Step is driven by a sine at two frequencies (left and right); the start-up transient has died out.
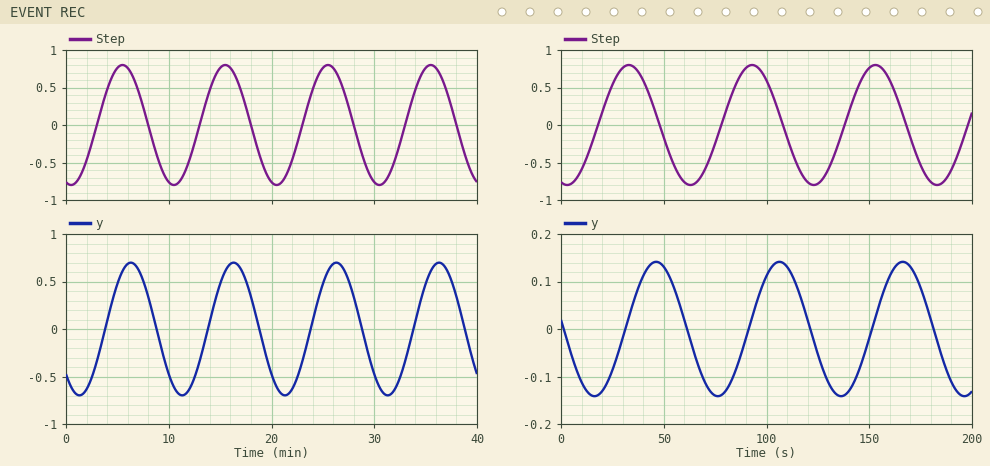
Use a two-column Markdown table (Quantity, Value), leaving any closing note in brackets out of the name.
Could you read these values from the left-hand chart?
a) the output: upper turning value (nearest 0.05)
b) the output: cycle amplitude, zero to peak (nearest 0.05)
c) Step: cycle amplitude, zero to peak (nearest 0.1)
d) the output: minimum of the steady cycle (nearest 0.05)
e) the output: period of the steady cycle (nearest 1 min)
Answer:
| Quantity | Value |
|---|---|
| the output: upper turning value | 0.70 |
| the output: cycle amplitude, zero to peak | 0.70 |
| Step: cycle amplitude, zero to peak | 0.8 |
| the output: minimum of the steady cycle | -0.70 |
| the output: period of the steady cycle | 10 min |
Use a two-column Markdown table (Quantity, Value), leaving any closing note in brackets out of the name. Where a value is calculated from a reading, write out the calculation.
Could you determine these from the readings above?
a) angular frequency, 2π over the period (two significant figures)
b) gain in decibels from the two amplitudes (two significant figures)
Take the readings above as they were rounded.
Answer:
| Quantity | Value |
|---|---|
| angular frequency, 2π over the period | 2π / 10 = 0.63 rad/min |
| gain in decibels from the two amplitudes | 20 log10(0.7 / 0.8) = -1.2 dB |
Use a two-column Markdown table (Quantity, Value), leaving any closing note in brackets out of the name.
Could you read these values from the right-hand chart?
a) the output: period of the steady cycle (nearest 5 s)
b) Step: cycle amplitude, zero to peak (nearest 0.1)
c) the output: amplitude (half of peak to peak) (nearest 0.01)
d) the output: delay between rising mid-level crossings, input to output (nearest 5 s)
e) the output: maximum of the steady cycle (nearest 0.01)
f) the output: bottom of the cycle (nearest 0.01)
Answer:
| Quantity | Value |
|---|---|
| the output: period of the steady cycle | 60 s |
| Step: cycle amplitude, zero to peak | 0.8 |
| the output: amplitude (half of peak to peak) | 0.14 |
| the output: delay between rising mid-level crossings, input to output | 15 s |
| the output: maximum of the steady cycle | 0.14 |
| the output: bottom of the cycle | -0.14 |
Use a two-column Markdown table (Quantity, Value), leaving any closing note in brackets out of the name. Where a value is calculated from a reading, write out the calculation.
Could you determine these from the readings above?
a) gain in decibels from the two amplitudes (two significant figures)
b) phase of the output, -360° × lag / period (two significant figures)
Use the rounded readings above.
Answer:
| Quantity | Value |
|---|---|
| gain in decibels from the two amplitudes | 20 log10(0.14 / 0.8) = -15 dB |
| phase of the output, -360° × lag / period | -360 × 15 / 60 = -90° |
